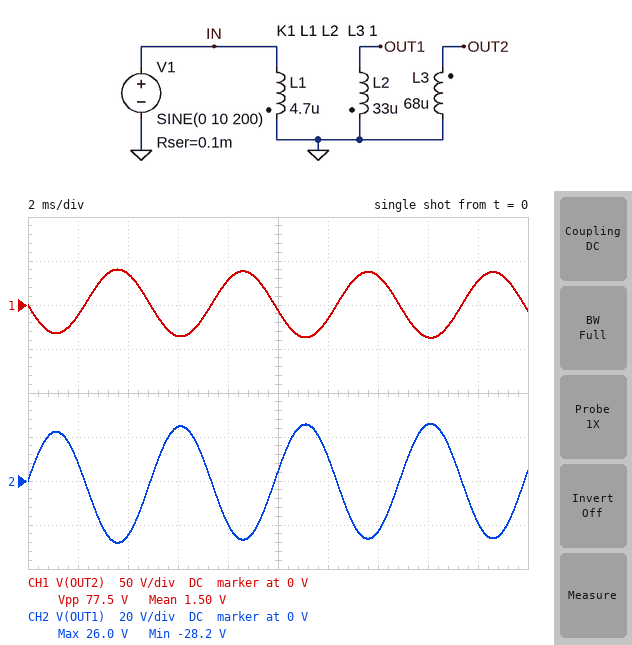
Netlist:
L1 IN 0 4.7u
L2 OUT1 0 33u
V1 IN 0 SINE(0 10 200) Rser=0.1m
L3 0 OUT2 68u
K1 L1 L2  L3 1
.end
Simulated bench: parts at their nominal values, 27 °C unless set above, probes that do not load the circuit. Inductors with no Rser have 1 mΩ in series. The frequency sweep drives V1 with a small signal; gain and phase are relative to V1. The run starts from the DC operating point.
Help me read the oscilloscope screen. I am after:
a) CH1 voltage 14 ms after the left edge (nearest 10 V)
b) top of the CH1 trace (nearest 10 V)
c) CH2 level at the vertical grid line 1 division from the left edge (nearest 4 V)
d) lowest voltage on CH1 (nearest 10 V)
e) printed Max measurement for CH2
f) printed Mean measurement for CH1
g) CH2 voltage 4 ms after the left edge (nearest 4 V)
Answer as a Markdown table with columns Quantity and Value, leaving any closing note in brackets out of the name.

| Quantity | Value |
|---|---|
| CH1 voltage 14 ms after the left edge | 30 V |
| top of the CH1 trace | 40 V |
| CH2 level at the vertical grid line 1 division from the left edge | 8 V |
| lowest voltage on CH1 | -40 V |
| printed Max measurement for CH2 | 26.0 V |
| printed Mean measurement for CH1 | 1.50 V |
| CH2 voltage 4 ms after the left edge | -24 V |
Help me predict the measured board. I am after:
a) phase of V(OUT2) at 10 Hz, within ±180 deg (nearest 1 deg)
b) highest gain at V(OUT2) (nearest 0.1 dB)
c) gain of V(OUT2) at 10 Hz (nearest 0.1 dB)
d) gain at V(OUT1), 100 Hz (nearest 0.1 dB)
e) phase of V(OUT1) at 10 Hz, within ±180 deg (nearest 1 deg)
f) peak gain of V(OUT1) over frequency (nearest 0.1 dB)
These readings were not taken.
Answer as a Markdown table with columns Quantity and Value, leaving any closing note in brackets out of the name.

| Quantity | Value |
|---|---|
| phase of V(OUT2) at 10 Hz, within ±180 deg | -105 deg |
| highest gain at V(OUT2) | 11.6 dB |
| gain of V(OUT2) at 10 Hz | -0.1 dB |
| gain at V(OUT1), 100 Hz | 7.9 dB |
| phase of V(OUT1) at 10 Hz, within ±180 deg | 75 deg |
| peak gain of V(OUT1) over frequency | 8.5 dB |
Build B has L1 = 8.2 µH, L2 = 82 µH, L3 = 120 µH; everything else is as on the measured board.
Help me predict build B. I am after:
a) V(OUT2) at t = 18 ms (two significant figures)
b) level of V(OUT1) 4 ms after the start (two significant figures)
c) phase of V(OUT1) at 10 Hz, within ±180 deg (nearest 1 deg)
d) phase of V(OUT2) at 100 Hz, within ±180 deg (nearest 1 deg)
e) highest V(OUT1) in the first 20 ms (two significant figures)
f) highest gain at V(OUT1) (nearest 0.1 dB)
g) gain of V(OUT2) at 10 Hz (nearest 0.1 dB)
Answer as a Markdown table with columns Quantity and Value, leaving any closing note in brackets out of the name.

| Quantity | Value |
|---|---|
| V(OUT2) at t = 18 ms | 26 V |
| level of V(OUT1) 4 ms after the start | -31 V |
| phase of V(OUT1) at 10 Hz, within ±180 deg | 65 deg |
| phase of V(OUT2) at 100 Hz, within ±180 deg | -168 deg |
| highest V(OUT1) in the first 20 ms | 31 V |
| highest gain at V(OUT1) | 10.0 dB |
| gain of V(OUT2) at 10 Hz | 4.2 dB |
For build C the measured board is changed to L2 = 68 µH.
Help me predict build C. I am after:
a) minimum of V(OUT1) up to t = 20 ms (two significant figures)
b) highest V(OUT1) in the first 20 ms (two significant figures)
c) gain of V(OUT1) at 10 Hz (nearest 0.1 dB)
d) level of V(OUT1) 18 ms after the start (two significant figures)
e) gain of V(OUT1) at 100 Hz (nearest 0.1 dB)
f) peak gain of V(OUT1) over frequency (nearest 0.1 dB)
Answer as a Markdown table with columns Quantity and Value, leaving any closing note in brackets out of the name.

| Quantity | Value |
|---|---|
| minimum of V(OUT1) up to t = 20 ms | -40 V |
| highest V(OUT1) in the first 20 ms | 37 V |
| gain of V(OUT1) at 10 Hz | -0.1 dB |
| level of V(OUT1) 18 ms after the start | -27 V |
| gain of V(OUT1) at 100 Hz | 11.0 dB |
| peak gain of V(OUT1) over frequency | 11.6 dB |
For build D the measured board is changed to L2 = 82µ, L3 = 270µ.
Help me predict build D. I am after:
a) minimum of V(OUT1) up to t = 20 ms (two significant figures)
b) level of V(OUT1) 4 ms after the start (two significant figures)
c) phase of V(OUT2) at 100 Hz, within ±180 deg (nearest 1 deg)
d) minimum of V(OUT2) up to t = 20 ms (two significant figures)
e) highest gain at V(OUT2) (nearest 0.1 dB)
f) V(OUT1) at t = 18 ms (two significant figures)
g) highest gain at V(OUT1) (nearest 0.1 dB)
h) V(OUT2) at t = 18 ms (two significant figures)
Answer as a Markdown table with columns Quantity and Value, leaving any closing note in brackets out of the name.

| Quantity | Value |
|---|---|
| minimum of V(OUT1) up to t = 20 ms | -44 V |
| level of V(OUT1) 4 ms after the start | -39 V |
| phase of V(OUT2) at 100 Hz, within ±180 deg | -160 deg |
| minimum of V(OUT2) up to t = 20 ms | -74 V |
| highest gain at V(OUT2) | 17.6 dB |
| V(OUT1) at t = 18 ms | -30 V |
| highest gain at V(OUT1) | 12.4 dB |
| V(OUT2) at t = 18 ms | 54 V |
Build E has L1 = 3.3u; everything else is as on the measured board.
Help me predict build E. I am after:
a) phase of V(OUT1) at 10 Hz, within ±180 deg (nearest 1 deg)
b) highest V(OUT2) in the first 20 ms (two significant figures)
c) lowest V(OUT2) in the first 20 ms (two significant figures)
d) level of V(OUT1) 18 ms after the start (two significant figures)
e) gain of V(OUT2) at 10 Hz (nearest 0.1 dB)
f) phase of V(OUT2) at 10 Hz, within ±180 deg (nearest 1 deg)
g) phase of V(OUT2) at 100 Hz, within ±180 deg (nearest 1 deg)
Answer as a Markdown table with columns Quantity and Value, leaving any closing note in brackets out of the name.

| Quantity | Value |
|---|---|
| phase of V(OUT1) at 10 Hz, within ±180 deg | 79 deg |
| highest V(OUT2) in the first 20 ms | 47 V |
| lowest V(OUT2) in the first 20 ms | -44 V |
| level of V(OUT1) 18 ms after the start | -24 V |
| gain of V(OUT2) at 10 Hz | -1.5 dB |
| phase of V(OUT2) at 10 Hz, within ±180 deg | -101 deg |
| phase of V(OUT2) at 100 Hz, within ±180 deg | -152 deg |
